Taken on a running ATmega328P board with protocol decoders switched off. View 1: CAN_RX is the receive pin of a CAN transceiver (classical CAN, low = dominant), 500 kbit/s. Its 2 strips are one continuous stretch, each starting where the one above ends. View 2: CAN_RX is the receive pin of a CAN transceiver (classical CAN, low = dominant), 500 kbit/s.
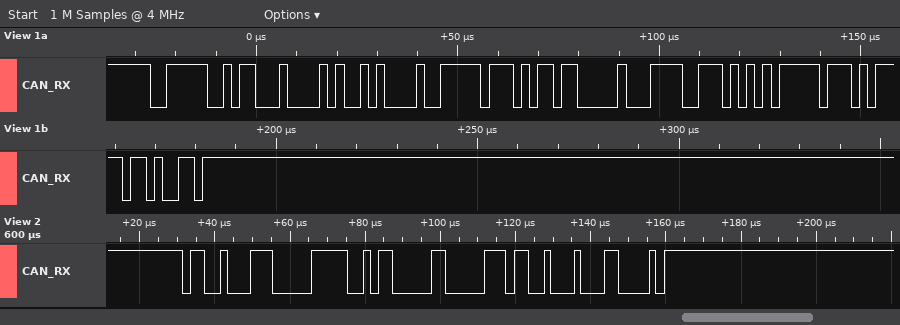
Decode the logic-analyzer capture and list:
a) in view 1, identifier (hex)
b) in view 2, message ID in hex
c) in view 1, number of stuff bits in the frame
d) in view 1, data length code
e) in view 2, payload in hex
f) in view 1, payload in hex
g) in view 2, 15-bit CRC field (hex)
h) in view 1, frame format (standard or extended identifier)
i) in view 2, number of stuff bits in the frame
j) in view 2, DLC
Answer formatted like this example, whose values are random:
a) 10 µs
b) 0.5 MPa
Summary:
a) 0x3EB
b) 0x647
c) 4
d) 8
e) D6 08 36
f) 52 84 FF 5B 00 F3 AA FF
g) 0x2230
h) standard
i) 4
j) 3
